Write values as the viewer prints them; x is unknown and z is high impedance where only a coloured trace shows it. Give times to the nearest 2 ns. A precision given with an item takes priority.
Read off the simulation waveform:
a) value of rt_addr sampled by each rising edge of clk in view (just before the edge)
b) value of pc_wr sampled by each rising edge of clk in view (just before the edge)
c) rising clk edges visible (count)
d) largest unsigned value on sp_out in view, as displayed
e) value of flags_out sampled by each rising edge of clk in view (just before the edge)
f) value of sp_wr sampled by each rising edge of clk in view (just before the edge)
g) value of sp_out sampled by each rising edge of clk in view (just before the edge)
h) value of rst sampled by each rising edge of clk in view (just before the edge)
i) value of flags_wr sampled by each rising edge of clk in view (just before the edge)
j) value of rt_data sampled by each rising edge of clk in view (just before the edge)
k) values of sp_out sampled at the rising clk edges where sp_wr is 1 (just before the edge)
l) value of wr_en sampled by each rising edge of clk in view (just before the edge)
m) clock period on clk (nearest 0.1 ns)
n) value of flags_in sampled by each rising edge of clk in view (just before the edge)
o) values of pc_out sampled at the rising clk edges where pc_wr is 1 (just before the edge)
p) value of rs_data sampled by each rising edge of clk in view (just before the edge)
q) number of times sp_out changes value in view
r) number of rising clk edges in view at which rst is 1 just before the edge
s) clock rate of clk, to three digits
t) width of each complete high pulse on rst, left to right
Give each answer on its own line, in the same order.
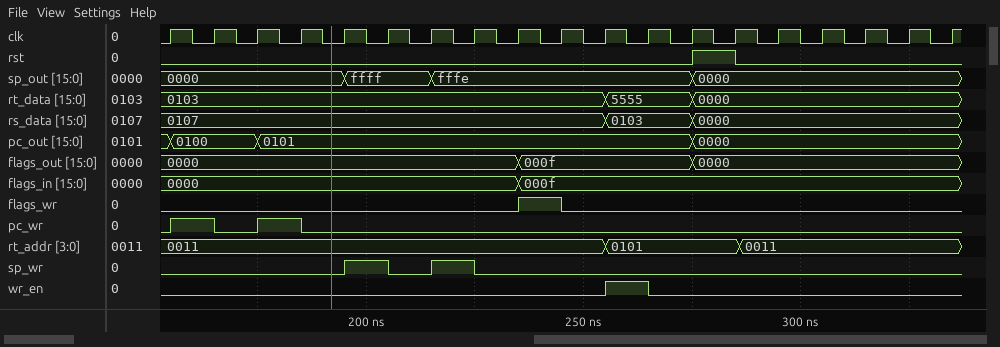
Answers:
0011, 0011, 0011, 0011, 0011, 0011, 0011, 0011, 0011, 0011, 0011, 0101, 0101, 0101, 0011, 0011, 0011, 0011, 0011
0 1 0 1 0 0 0 0 0 0 0 0 0 0 0 0 0 0 0
19
ffff
0000, 0000, 0000, 0000, 0000, 0000, 0000, 0000, 0000, 000f, 000f, 000f, 000f, 0000, 0000, 0000, 0000, 0000, 0000
0 0 0 0 0 1 0 1 0 0 0 0 0 0 0 0 0 0 0
0000, 0000, 0000, 0000, 0000, ffff, ffff, fffe, fffe, fffe, fffe, fffe, fffe, 0000, 0000, 0000, 0000, 0000, 0000
0 0 0 0 0 0 0 0 0 0 0 0 0 1 0 0 0 0 0
0 0 0 0 0 0 0 0 0 1 0 0 0 0 0 0 0 0 0
0103, 0103, 0103, 0103, 0103, 0103, 0103, 0103, 0103, 0103, 0103, 5555, 5555, 0000, 0000, 0000, 0000, 0000, 0000
ffff, fffe
0 0 0 0 0 0 0 0 0 0 0 1 0 0 0 0 0 0 0
10 ns
0000, 0000, 0000, 0000, 0000, 0000, 0000, 0000, 0000, 000f, 000f, 000f, 000f, 000f, 000f, 000f, 000f, 000f, 000f
0100, 0101
0107, 0107, 0107, 0107, 0107, 0107, 0107, 0107, 0107, 0107, 0107, 0103, 0103, 0000, 0000, 0000, 0000, 0000, 0000
3
1
100 MHz
10 ns
